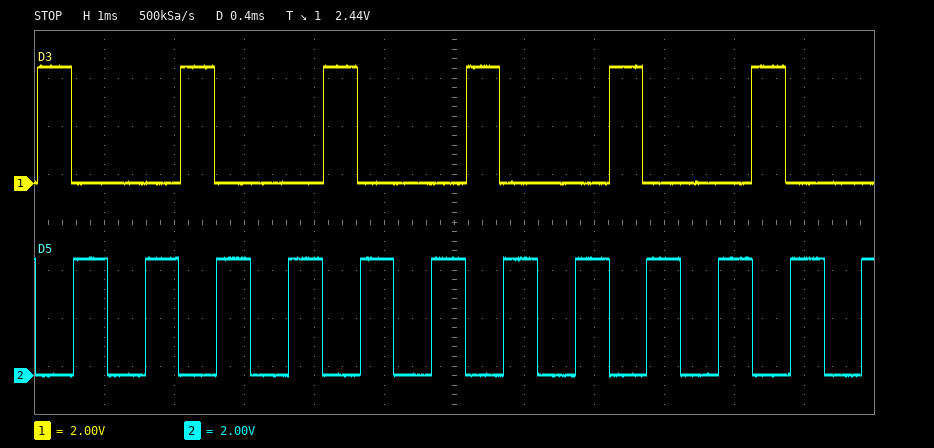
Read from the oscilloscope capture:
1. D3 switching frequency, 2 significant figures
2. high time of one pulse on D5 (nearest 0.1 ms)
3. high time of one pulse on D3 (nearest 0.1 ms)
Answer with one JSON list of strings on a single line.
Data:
["490 Hz", "0.5 ms", "0.5 ms"]
